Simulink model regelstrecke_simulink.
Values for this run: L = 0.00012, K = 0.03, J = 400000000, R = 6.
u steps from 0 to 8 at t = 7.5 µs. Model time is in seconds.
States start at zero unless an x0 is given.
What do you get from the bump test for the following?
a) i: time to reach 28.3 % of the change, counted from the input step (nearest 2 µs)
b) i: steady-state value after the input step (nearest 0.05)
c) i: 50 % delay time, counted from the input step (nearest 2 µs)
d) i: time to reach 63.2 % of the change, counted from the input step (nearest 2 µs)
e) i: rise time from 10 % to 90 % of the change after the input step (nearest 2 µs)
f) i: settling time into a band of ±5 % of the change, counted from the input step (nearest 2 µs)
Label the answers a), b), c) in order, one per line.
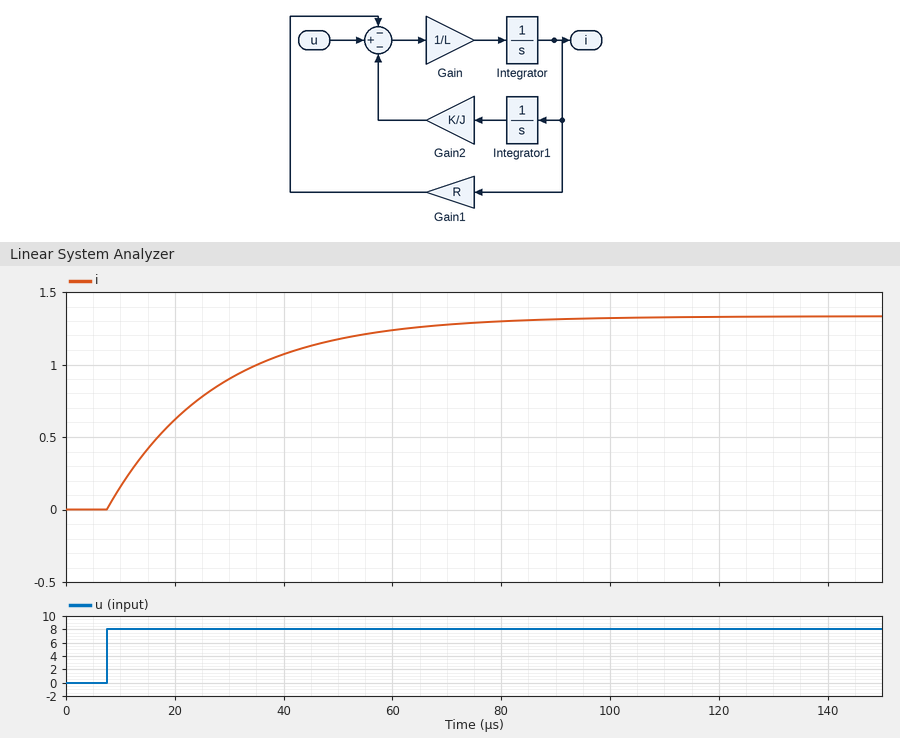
a) 6 µs
b) 1.35
c) 14 µs
d) 20 µs
e) 44 µs
f) 60 µs
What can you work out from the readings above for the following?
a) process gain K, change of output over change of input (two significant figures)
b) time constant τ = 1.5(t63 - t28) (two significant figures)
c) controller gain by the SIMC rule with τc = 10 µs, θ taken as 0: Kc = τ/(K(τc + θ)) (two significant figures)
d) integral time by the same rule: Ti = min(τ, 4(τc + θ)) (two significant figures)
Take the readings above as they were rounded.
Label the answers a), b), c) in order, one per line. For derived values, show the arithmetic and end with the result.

a) (1.35 - 0) / 8 = 0.17
b) 1.5 × (20 - 6) = 21 µs
c) 21 / (0.17 × (10 + 0)) = 12
d) min(21, 4 × (10 + 0)) = 21 µs
